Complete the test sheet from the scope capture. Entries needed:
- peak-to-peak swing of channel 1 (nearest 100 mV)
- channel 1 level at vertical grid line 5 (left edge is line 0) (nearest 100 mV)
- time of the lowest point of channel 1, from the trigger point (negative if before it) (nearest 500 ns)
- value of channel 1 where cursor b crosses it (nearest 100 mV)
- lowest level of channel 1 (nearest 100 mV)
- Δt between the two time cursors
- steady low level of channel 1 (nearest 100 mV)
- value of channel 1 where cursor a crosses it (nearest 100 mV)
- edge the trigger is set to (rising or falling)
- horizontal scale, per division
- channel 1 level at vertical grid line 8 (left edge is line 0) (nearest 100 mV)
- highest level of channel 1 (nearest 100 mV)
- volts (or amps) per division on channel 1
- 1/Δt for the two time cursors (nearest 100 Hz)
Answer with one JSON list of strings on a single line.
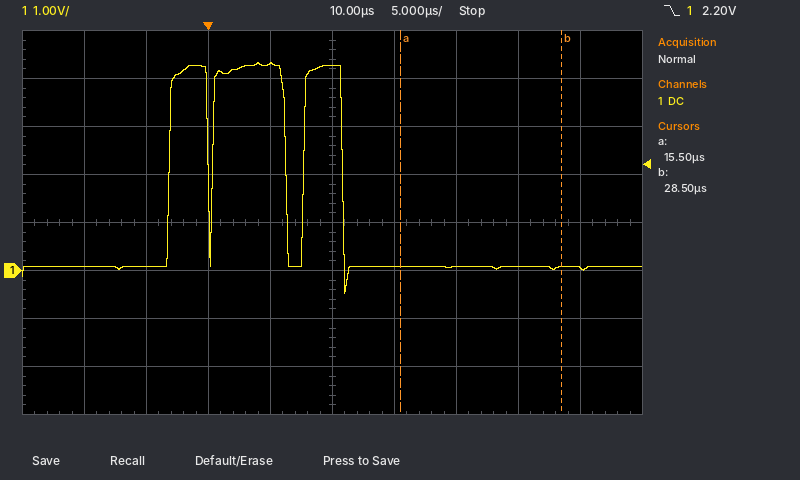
["4.8 V", "4.3 V", "+11.0 µs", "100 mV", "-500 mV", "13.0 µs", "100 mV", "100 mV", "falling", "5 µs", "100 mV", "4.3 V", "1 V", "76.9 kHz"]
